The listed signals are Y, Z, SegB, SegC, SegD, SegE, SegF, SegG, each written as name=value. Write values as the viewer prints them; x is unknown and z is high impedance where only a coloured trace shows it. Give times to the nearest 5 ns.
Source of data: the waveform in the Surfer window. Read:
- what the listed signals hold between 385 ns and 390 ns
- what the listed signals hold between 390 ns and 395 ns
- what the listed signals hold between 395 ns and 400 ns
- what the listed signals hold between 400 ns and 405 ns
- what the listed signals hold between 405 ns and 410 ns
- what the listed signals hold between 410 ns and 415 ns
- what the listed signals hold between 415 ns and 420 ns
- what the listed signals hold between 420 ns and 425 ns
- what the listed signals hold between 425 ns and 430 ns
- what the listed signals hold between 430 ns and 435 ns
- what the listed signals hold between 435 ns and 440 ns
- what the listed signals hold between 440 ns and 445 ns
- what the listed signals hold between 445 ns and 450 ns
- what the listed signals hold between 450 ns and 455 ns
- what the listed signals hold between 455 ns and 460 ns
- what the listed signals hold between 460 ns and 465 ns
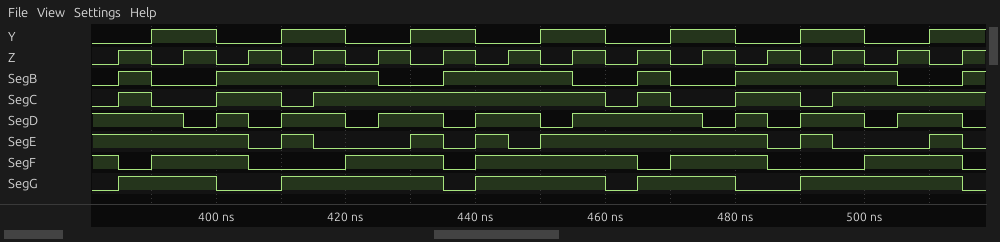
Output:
Y=0, Z=1, SegB=1, SegC=1, SegD=1, SegE=1, SegF=0, SegG=1
Y=1, Z=0, SegB=0, SegC=0, SegD=1, SegE=1, SegF=1, SegG=1
Y=1, Z=1, SegB=0, SegC=0, SegD=0, SegE=1, SegF=1, SegG=1
Y=0, Z=0, SegB=1, SegC=1, SegD=1, SegE=1, SegF=1, SegG=0
Y=0, Z=1, SegB=1, SegC=1, SegD=0, SegE=0, SegF=0, SegG=0
Y=1, Z=0, SegB=1, SegC=0, SegD=1, SegE=1, SegF=0, SegG=1
Y=1, Z=1, SegB=1, SegC=1, SegD=1, SegE=0, SegF=0, SegG=1
Y=0, Z=0, SegB=1, SegC=1, SegD=0, SegE=0, SegF=1, SegG=1
Y=0, Z=1, SegB=0, SegC=1, SegD=1, SegE=0, SegF=1, SegG=1
Y=1, Z=0, SegB=0, SegC=1, SegD=1, SegE=1, SegF=1, SegG=1
Y=1, Z=1, SegB=1, SegC=1, SegD=0, SegE=0, SegF=0, SegG=0
Y=0, Z=0, SegB=1, SegC=1, SegD=1, SegE=1, SegF=1, SegG=1
Y=0, Z=1, SegB=1, SegC=1, SegD=1, SegE=0, SegF=1, SegG=1
Y=1, Z=0, SegB=1, SegC=1, SegD=0, SegE=1, SegF=1, SegG=1
Y=1, Z=1, SegB=0, SegC=1, SegD=1, SegE=1, SegF=1, SegG=1
Y=0, Z=0, SegB=0, SegC=0, SegD=1, SegE=1, SegF=1, SegG=0
